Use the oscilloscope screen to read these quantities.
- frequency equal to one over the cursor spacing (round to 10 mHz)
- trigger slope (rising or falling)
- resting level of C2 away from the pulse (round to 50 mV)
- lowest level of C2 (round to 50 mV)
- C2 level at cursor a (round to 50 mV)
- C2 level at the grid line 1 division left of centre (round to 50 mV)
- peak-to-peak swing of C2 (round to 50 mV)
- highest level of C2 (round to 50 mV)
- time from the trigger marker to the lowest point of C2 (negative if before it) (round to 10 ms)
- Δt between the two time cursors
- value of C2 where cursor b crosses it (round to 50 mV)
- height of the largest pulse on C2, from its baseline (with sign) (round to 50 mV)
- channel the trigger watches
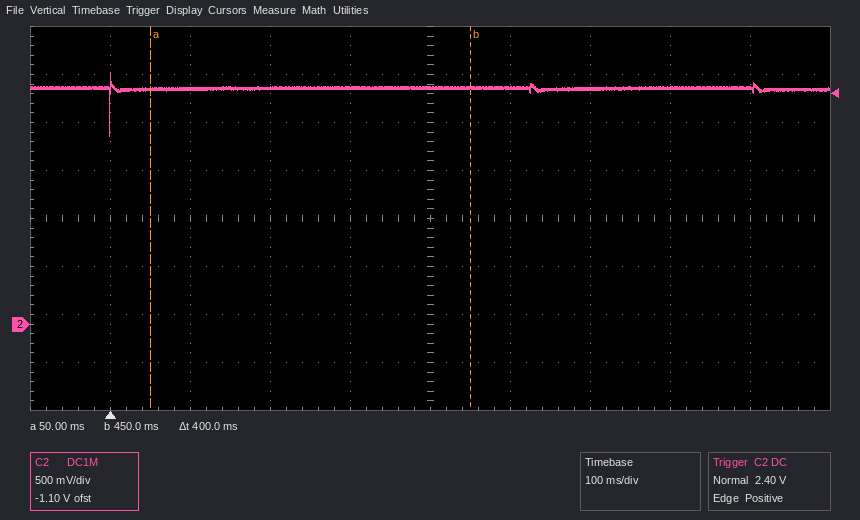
2.50 Hz
rising
2.45 V
1.95 V
2.45 V
2.45 V
650 mV
2.60 V
0 ms
400 ms
2.45 V
-500 mV
C2
